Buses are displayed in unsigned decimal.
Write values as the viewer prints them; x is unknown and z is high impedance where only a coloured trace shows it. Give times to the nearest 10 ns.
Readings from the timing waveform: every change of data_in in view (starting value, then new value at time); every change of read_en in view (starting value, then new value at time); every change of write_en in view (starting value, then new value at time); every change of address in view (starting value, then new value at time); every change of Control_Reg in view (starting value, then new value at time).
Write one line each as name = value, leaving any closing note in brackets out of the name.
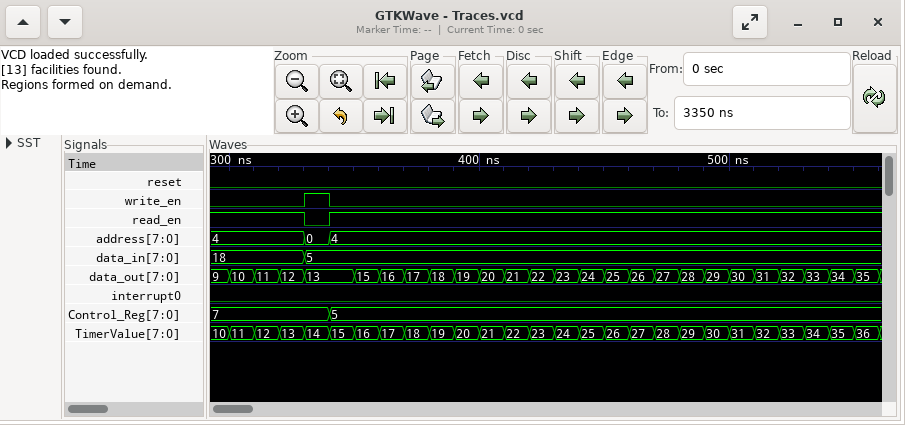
every change of data_in in view = 18, 5 at 330 ns
every change of read_en in view = 1, 0 at 330 ns, 1 at 340 ns
every change of write_en in view = 0, 1 at 330 ns, 0 at 340 ns
every change of address in view = 4, 0 at 330 ns, 4 at 340 ns
every change of Control_Reg in view = 7, 5 at 340 ns
